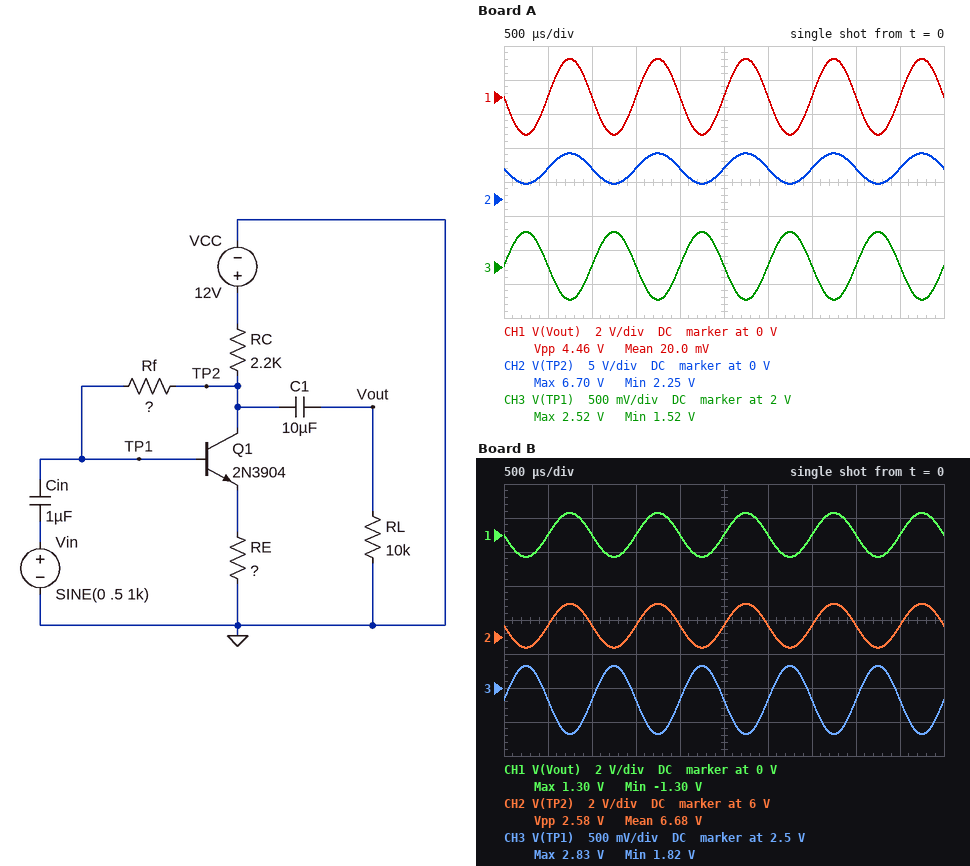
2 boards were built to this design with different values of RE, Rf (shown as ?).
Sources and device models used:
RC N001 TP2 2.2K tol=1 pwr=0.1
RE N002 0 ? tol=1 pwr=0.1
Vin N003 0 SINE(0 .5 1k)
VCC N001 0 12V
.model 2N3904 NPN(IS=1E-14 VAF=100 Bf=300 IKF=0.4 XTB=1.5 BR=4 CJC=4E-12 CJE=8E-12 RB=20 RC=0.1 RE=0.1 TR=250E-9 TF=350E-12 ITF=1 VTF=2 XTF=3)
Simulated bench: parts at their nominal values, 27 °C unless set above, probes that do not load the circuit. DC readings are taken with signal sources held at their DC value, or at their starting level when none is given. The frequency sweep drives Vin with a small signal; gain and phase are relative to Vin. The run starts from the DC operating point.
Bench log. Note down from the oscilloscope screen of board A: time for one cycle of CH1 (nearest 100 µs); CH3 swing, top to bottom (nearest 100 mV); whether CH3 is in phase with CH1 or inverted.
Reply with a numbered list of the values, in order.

1. 1.0 ms
2. 1.0 V
3. inverted
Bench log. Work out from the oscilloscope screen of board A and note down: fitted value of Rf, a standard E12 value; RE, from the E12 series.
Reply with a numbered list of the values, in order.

1. 220 kΩ
2. 390 Ω
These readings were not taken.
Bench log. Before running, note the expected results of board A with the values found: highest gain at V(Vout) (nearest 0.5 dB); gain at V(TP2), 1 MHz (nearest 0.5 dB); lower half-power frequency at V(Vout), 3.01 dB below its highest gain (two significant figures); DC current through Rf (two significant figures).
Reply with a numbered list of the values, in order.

1. 13.0 dB
2. 13.0 dB
3. 5.5 Hz
4. 11 µA
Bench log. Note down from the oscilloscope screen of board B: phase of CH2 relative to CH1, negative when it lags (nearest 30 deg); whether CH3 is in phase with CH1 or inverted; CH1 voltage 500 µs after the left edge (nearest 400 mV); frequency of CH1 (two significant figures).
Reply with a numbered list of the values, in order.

1. 0 deg
2. inverted
3. 0 V
4. 1.0 kHz
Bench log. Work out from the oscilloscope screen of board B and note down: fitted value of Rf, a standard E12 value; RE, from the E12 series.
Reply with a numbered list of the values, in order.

1. 560 kΩ
2. 680 Ω
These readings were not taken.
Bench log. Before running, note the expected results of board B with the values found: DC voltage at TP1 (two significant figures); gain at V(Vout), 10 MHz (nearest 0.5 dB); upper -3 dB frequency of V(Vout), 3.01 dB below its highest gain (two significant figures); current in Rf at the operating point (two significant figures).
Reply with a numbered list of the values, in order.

1. 2.3 V
2. 8.0 dB
3. 52 MHz
4. 7.8 µA
